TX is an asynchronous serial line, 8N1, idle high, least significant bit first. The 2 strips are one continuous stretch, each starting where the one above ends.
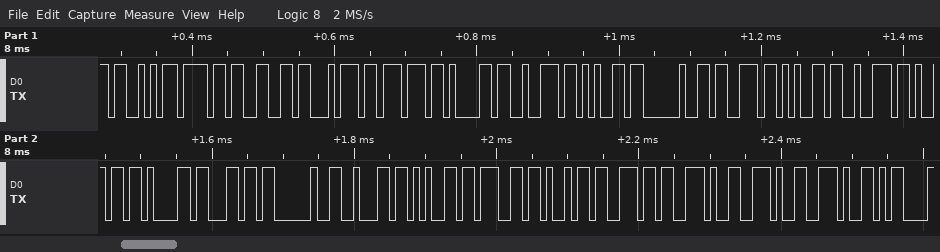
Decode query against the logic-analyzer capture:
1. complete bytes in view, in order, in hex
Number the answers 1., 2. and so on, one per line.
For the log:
1. 0x53 0x6F 0x66 0x74 0x77 0x61 0x72 0x65 0x20 0x73 0x65 0x72 0x69 0x61 0x6C 0x20 0x62 0x65 0x67 0x69 0x6E 0x2E 0x2E 0x2E 0x0D
